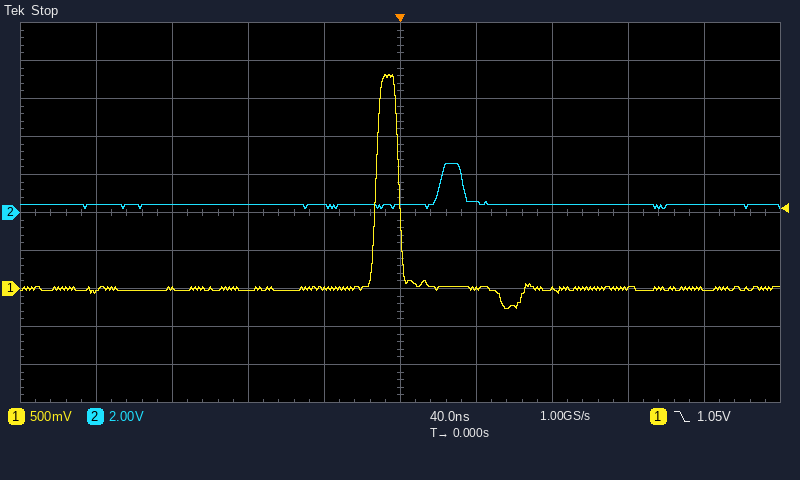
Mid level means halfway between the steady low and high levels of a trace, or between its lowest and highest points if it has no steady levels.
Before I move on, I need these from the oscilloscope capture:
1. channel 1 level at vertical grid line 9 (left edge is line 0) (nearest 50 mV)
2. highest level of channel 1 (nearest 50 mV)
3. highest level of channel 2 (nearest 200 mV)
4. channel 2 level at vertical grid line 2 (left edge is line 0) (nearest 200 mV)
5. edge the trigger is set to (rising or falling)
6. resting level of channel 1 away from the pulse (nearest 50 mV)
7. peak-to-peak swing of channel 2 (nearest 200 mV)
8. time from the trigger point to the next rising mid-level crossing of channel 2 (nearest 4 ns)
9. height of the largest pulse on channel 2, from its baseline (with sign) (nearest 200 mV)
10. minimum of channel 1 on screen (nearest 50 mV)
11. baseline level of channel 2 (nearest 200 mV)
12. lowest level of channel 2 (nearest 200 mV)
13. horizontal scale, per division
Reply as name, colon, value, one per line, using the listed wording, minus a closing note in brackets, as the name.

channel 1 level at vertical grid line 9 (left edge is line 0): 0 mV
highest level of channel 1: 2.80 V
highest level of channel 2: 2.6 V
channel 2 level at vertical grid line 2 (left edge is line 0): 400 mV
edge the trigger is set to: falling
resting level of channel 1 away from the pulse: 0 mV
peak-to-peak swing of channel 2: 2.4 V
time from the trigger point to the next rising mid-level crossing of channel 2: 20 ns
height of the largest pulse on channel 2, from its baseline (with sign): +2.2 V
minimum of channel 1 on screen: -250 mV
baseline level of channel 2: 400 mV
lowest level of channel 2: 200 mV
horizontal scale, per division: 40 ns
